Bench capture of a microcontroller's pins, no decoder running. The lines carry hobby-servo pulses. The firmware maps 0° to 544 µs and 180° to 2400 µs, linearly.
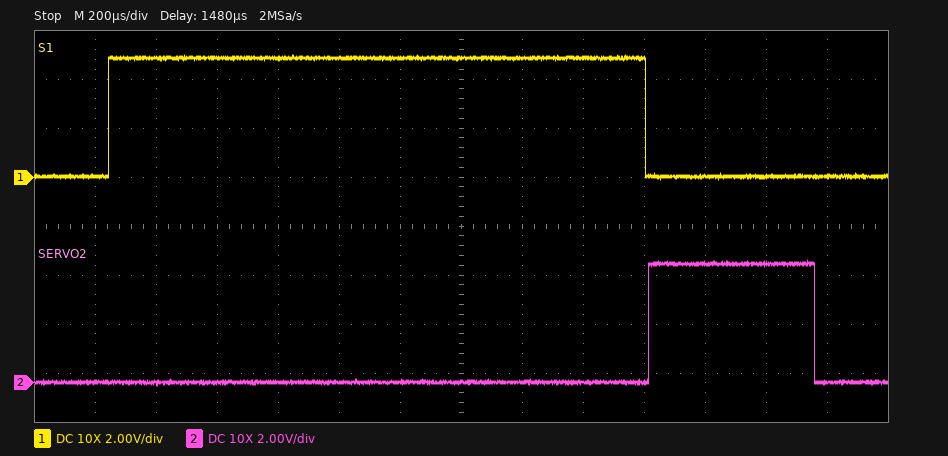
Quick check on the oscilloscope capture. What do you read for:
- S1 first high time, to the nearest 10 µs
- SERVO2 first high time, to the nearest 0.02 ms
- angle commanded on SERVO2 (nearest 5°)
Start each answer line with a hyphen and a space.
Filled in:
- 1760 µs
- 0.54 ms
- 0°
